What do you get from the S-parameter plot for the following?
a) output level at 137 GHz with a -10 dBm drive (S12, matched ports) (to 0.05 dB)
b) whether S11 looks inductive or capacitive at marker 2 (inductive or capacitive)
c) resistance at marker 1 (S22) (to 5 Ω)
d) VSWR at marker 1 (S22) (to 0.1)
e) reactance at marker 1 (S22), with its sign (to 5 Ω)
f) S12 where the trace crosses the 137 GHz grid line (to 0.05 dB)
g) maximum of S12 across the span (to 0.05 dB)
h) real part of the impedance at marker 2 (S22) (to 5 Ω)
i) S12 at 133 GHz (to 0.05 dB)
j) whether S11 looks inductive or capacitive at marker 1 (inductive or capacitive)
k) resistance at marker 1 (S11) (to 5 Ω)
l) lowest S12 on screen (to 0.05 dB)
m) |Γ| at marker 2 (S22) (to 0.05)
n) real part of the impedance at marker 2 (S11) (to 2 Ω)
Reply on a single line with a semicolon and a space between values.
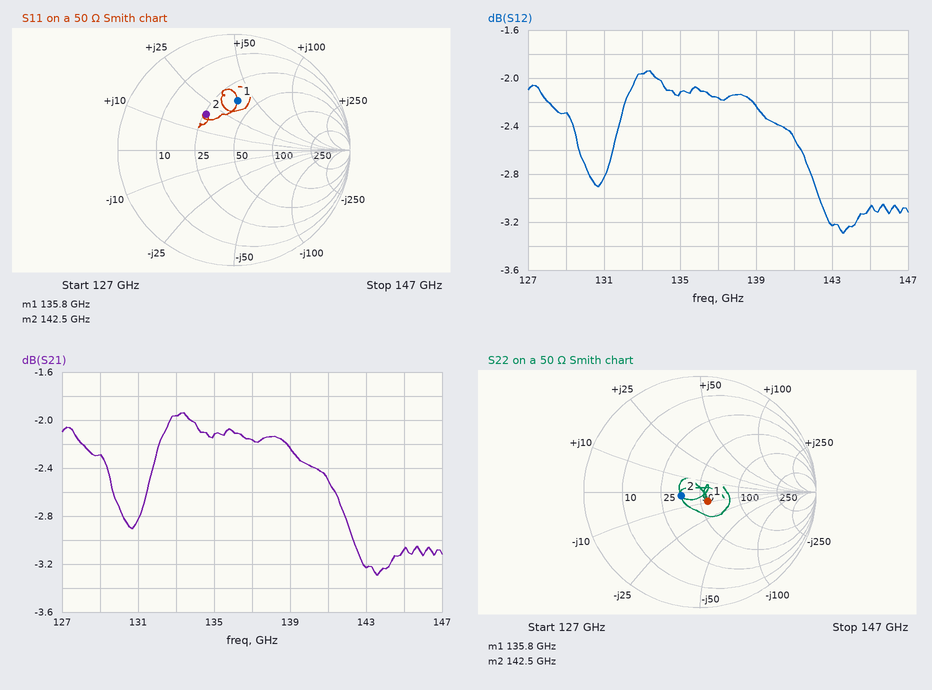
-12.15 dBm; inductive; 55 Ω; 1.2; -10 Ω; -2.15 dB; -1.95 dB; 35 Ω; -1.95 dB; inductive; 35 Ω; -3.30 dB; 0.15; 26 Ω
